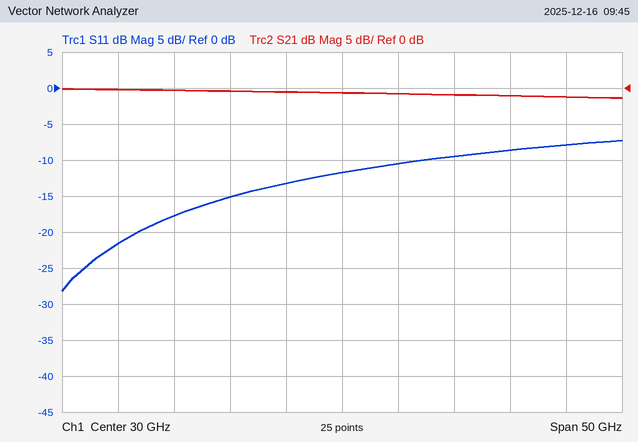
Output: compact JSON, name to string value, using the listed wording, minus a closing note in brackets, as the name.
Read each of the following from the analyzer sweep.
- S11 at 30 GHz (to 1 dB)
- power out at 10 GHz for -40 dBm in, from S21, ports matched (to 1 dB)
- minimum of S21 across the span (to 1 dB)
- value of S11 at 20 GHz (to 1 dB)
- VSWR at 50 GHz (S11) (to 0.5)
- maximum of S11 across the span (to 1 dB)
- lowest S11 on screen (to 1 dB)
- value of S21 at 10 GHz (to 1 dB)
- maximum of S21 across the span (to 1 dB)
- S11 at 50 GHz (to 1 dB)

{"S11 at 30 GHz": "-12 dB", "power out at 10 GHz for -40 dBm in, from S21, ports matched": "-40 dBm", "minimum of S21 across the span": "-1 dB", "value of S11 at 20 GHz": "-15 dB", "VSWR at 50 GHz (S11)": "2.5", "maximum of S11 across the span": "-7 dB", "lowest S11 on screen": "-28 dB", "value of S21 at 10 GHz": "0 dB", "maximum of S21 across the span": "0 dB", "S11 at 50 GHz": "-8 dB"}
